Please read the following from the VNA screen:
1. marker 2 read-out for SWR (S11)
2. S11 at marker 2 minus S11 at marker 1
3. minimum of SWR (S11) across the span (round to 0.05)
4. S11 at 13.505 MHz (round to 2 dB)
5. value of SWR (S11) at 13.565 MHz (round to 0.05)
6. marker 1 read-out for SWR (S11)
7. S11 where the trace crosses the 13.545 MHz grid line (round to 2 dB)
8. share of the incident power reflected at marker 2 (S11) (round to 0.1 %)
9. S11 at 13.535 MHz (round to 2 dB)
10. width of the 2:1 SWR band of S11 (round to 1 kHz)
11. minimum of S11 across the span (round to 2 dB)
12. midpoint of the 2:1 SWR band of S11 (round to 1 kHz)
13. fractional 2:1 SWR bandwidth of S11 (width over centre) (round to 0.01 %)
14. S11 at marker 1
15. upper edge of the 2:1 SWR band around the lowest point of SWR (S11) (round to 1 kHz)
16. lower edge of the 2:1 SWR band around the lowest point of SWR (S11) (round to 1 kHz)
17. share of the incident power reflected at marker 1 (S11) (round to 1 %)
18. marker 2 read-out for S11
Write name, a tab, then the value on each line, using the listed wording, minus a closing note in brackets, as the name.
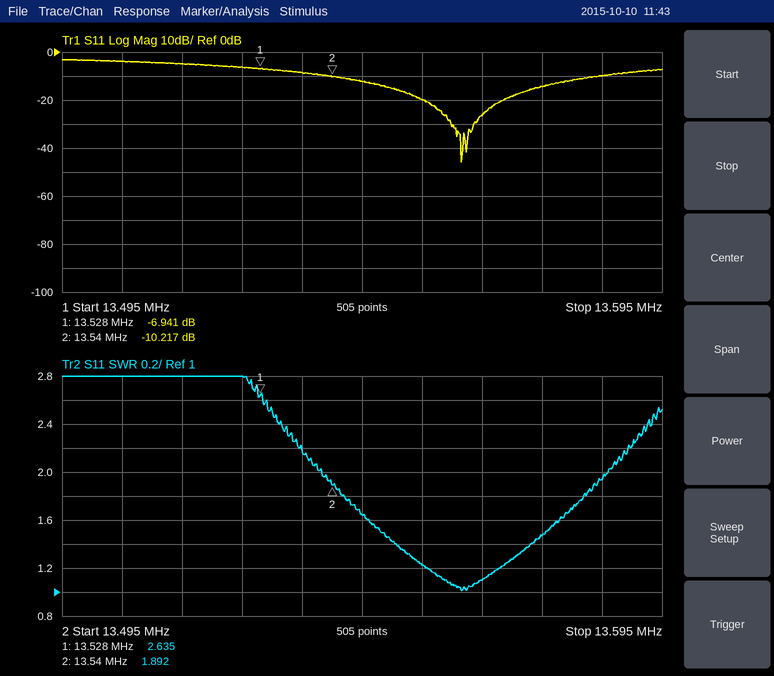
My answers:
marker 2 read-out for SWR	1.892
S11 at marker 2 minus S11 at marker 1	-3.276 dB
minimum of SWR (S11) across the span	1.00
S11 at 13.505 MHz	-4 dB
value of SWR (S11) at 13.565 MHz	1.10
marker 1 read-out for SWR	2.635
S11 where the trace crosses the 13.545 MHz grid line	-12 dB
share of the incident power reflected at marker 2 (S11)	9.5 %
S11 at 13.535 MHz	-8 dB
width of the 2:1 SWR band of S11	48 kHz
minimum of S11 across the span	-46 dB
midpoint of the 2:1 SWR band of S11	13.562 MHz
fractional 2:1 SWR bandwidth of S11 (width over centre)	0.35 %
S11 at marker 1	-6.941 dB
upper edge of the 2:1 SWR band around the lowest point of SWR (S11)	13.586 MHz
lower edge of the 2:1 SWR band around the lowest point of SWR (S11)	13.538 MHz
share of the incident power reflected at marker 1 (S11)	20 %
marker 2 read-out for S11	-10.217 dB
